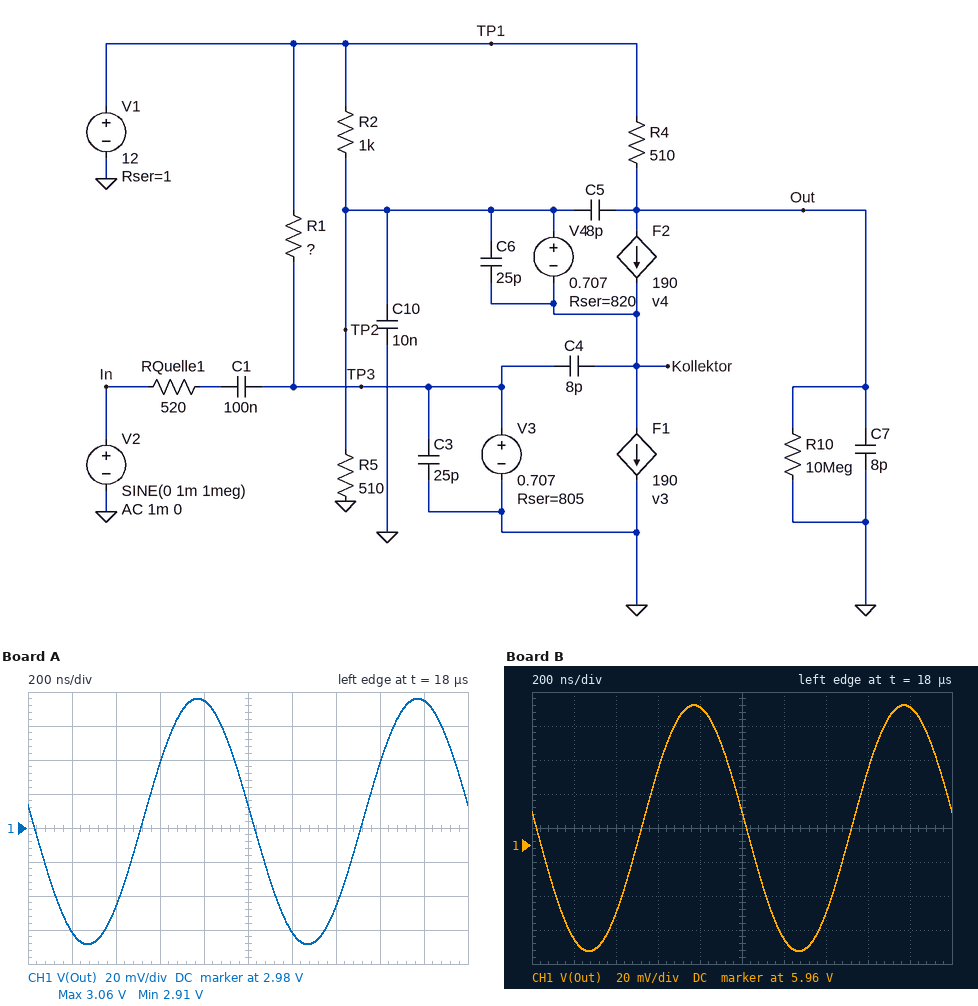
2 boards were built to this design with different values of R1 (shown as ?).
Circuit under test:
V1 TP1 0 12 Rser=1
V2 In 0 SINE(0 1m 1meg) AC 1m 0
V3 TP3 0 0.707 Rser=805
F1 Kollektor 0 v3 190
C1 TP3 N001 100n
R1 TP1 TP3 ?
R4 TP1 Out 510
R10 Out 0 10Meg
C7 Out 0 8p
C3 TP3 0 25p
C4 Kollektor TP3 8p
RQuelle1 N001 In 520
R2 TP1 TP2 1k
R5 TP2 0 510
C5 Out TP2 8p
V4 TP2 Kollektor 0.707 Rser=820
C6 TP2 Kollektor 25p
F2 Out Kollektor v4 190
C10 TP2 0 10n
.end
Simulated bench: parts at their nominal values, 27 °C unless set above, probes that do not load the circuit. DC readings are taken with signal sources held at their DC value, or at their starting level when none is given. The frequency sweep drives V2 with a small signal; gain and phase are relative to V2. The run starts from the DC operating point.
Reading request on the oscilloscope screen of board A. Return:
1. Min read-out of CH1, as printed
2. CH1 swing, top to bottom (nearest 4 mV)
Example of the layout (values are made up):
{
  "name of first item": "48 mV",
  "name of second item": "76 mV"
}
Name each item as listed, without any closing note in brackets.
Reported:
{
  "Min read-out of CH1, as printed": "2.91 V",
  "CH1 swing, top to bottom": "144 mV"
}
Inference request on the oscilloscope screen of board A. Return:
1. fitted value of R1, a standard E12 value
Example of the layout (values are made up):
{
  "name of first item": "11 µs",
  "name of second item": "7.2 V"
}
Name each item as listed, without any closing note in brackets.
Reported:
{
  "fitted value of R1, a standard E12 value": "120 kΩ"
}
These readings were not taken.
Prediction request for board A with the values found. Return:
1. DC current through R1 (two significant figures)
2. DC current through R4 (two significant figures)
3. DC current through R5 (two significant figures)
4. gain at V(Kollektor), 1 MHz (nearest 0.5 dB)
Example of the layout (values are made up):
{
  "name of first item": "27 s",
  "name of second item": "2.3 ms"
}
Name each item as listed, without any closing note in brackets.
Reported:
{
  "DC current through R1": "93 µA",
  "DC current through R4": "18 mA",
  "DC current through R5": "7.9 mA",
  "gain at V(Kollektor), 1 MHz": "-3.5 dB"
}
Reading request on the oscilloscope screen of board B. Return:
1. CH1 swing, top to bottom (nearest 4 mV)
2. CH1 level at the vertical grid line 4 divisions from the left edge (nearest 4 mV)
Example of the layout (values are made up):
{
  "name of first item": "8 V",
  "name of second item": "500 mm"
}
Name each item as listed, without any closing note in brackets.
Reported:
{
  "CH1 swing, top to bottom": "144 mV",
  "CH1 level at the vertical grid line 4 divisions from the left edge": "6.040 V"
}
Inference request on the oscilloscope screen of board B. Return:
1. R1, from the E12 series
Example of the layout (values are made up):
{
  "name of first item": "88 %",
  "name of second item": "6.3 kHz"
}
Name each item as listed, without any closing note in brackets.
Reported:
{
  "R1, from the E12 series": "180 kΩ"
}
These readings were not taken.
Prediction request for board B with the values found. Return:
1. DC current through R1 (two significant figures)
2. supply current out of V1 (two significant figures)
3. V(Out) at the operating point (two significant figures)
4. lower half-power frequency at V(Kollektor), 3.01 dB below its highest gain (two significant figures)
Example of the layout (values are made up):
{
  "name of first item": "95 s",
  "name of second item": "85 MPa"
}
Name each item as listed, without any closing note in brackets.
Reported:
{
  "DC current through R1": "62 µA",
  "supply current out of V1": "20 mA",
  "V(Out) at the operating point": "6.0 V",
  "lower half-power frequency at V(Kollektor), 3.01 dB below its highest gain": "1.2 kHz"
}
